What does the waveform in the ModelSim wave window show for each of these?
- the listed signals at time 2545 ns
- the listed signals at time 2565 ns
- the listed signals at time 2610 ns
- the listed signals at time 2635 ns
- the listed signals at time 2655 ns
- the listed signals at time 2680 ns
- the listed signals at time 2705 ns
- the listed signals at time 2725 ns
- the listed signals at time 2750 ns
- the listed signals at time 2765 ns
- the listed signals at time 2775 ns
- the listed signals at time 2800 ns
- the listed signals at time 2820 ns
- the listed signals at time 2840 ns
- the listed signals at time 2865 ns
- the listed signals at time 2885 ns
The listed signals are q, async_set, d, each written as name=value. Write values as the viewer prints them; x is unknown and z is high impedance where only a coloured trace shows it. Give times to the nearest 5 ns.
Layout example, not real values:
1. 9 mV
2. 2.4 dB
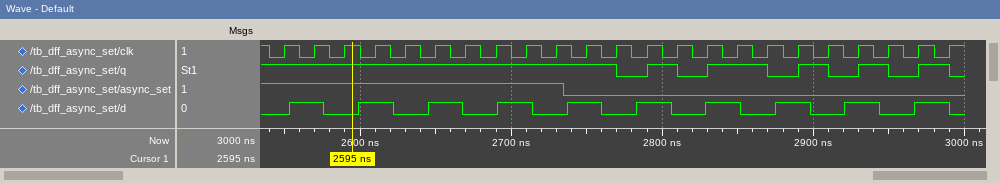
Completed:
1. q=1, async_set=1, d=0
2. q=1, async_set=1, d=1
3. q=1, async_set=1, d=1
4. q=1, async_set=1, d=0
5. q=1, async_set=1, d=1
6. q=1, async_set=1, d=0
7. q=1, async_set=1, d=1
8. q=1, async_set=1, d=0
9. q=1, async_set=0, d=1
10. q=1, async_set=0, d=0
11. q=0, async_set=0, d=0
12. q=1, async_set=0, d=1
13. q=0, async_set=0, d=0
14. q=1, async_set=0, d=1
15. q=1, async_set=0, d=0
16. q=0, async_set=0, d=1
